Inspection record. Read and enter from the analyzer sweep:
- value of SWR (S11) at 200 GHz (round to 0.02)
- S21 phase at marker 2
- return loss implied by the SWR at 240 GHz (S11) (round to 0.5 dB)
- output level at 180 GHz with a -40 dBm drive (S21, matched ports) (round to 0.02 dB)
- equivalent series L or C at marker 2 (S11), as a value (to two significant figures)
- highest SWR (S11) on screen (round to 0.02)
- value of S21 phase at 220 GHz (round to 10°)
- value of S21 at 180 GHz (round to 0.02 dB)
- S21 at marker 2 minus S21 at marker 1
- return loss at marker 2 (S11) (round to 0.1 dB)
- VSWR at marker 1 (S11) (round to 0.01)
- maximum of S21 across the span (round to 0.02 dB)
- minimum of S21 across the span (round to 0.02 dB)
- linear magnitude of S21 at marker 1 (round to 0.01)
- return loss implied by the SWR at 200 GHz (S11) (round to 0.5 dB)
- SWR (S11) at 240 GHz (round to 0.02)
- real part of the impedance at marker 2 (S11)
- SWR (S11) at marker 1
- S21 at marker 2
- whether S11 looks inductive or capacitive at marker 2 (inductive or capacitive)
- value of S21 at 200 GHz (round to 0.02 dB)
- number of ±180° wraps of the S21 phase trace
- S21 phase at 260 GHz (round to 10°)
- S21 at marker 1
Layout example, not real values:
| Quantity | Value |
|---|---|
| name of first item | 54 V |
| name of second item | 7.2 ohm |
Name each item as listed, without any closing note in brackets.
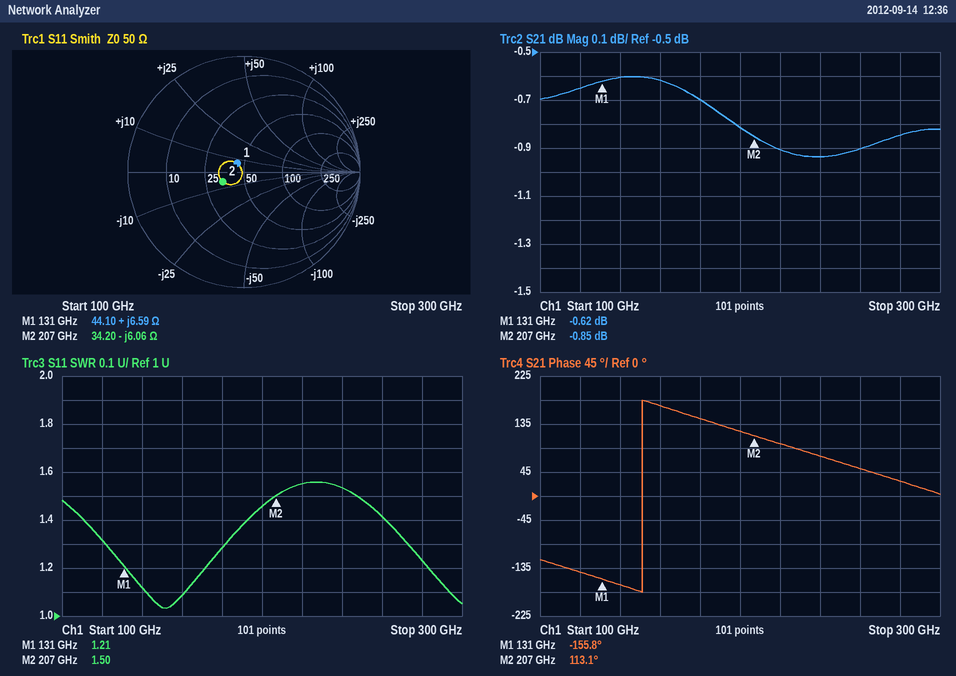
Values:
| Quantity | Value |
|---|---|
| value of SWR (S11) at 200 GHz | 1.46 |
| S21 phase at marker 2 | 113.1° |
| return loss implied by the SWR at 240 GHz (S11) | 13.5 dB |
| output level at 180 GHz with a -40 dBm drive (S21, matched ports) | -40.70 dBm |
| equivalent series L or C at marker 2 (S11), as a value | 130 fF |
| highest SWR (S11) on screen | 1.56 |
| value of S21 phase at 220 GHz | 100° |
| value of S21 at 180 GHz | -0.70 dB |
| S21 at marker 2 minus S21 at marker 1 | -0.23 dB |
| return loss at marker 2 (S11) | 14.0 dB |
| VSWR at marker 1 (S11) | 1.21 |
| maximum of S21 across the span | -0.60 dB |
| minimum of S21 across the span | -0.94 dB |
| linear magnitude of S21 at marker 1 | 0.93 |
| return loss implied by the SWR at 200 GHz (S11) | 14.5 dB |
| SWR (S11) at 240 GHz | 1.54 |
| real part of the impedance at marker 2 | 34.20 Ω |
| SWR (S11) at marker 1 | 1.21 |
| S21 at marker 2 | -0.85 dB |
| whether S11 looks inductive or capacitive at marker 2 | capacitive |
| value of S21 at 200 GHz | -0.82 dB |
| number of ±180° wraps of the S21 phase trace | 1 |
| S21 phase at 260 GHz | 50° |
| S21 at marker 1 | -0.62 dB |
